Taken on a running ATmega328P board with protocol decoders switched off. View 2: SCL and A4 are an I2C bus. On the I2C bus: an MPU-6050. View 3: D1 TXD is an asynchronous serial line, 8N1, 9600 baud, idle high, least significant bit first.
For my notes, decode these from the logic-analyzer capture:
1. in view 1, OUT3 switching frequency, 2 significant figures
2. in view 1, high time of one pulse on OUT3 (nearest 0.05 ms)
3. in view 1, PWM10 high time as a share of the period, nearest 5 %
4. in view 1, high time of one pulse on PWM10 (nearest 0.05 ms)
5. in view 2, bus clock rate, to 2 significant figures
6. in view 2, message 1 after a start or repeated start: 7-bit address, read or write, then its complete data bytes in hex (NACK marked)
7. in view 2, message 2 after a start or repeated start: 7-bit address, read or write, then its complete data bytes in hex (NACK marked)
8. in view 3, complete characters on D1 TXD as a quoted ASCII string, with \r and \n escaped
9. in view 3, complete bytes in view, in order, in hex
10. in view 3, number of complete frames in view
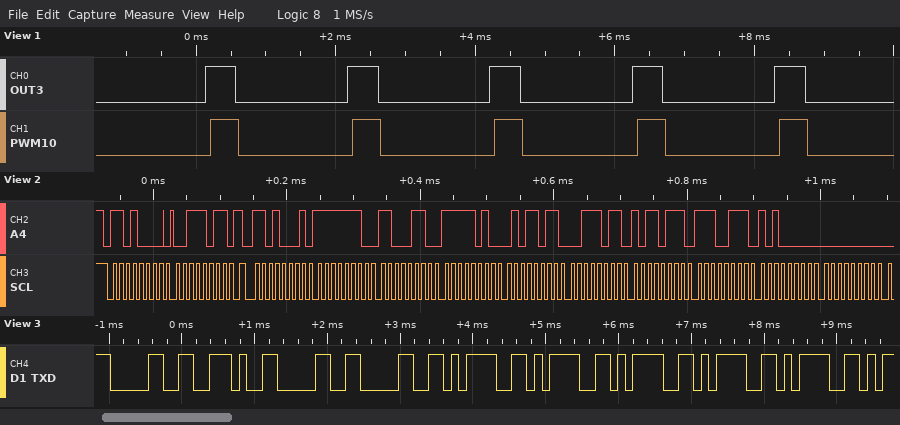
490 Hz
0.45 ms
20 %
0.40 ms
100 kHz
0x68 write: 3B
0x68 read: FE C6 FA 5B 3B B7 E7 A0 00
"0.00====="
0x30 0x2E 0x30 0x30 0x3D 0x3D 0x3D 0x3D 0x3D
9
